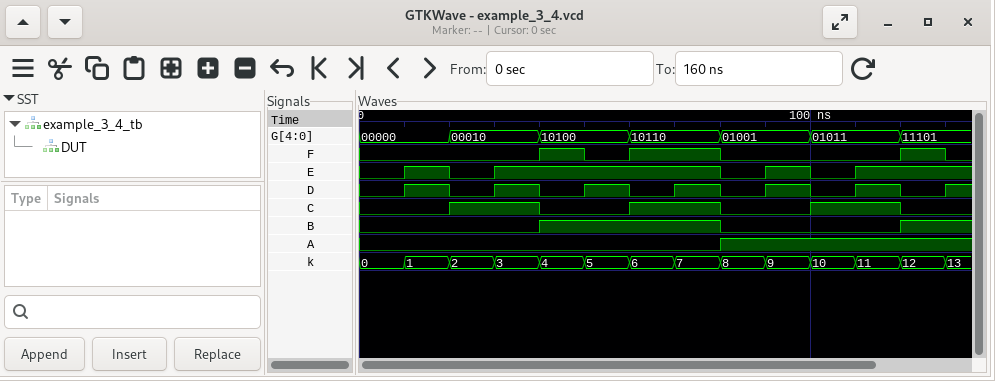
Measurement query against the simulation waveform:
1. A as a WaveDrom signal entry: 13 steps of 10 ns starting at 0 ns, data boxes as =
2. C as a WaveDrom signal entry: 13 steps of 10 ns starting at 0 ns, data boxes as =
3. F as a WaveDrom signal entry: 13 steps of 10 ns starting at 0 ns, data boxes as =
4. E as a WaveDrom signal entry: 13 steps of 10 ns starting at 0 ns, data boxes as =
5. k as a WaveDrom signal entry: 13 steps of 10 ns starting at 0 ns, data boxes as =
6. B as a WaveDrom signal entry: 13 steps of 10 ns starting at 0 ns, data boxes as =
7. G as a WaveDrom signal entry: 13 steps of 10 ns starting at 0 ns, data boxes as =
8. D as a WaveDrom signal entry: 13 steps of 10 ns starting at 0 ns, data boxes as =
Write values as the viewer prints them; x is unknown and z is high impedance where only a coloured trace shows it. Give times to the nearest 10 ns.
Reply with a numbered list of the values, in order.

1. {name: 'A', wave: '0.......1....'}
2. {name: 'C', wave: '0.1.0.1.0.1.0'}
3. {name: 'F', wave: '0...101.0...1'}
4. {name: 'E', wave: '0101....0101.'}
5. {name: 'k', wave: '=============', data: '0 1 2 3 4 5 6 7 8 9 10 11 12'}
6. {name: 'B', wave: '0...1...0...1'}
7. {name: 'G', wave: '=.=.=.=.=.=.=', data: '00000 00010 10100 10110 01001 01011 11101'}
8. {name: 'D', wave: '0101010101010'}
